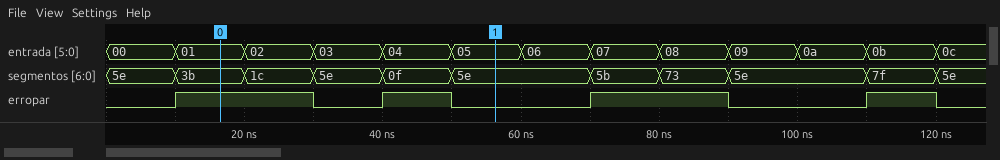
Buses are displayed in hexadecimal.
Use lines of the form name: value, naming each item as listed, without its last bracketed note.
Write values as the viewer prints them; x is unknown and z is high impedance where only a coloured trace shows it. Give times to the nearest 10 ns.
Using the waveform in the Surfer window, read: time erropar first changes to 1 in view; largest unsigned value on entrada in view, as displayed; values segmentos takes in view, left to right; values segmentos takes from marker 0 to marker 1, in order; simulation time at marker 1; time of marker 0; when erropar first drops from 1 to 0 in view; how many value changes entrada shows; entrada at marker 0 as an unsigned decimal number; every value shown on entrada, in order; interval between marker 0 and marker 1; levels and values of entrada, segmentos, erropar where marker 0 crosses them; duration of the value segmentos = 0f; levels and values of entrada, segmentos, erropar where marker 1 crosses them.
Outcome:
time erropar first changes to 1 in view: 10 ns
largest unsigned value on entrada in view, as displayed: 0c
values segmentos takes in view, left to right: 5e, 3b, 1c, 5e, 0f, 5e, 5b, 73, 5e, 7f, 5e
values segmentos takes from marker 0 to marker 1, in order: 3b, 1c, 5e, 0f, 5e
simulation time at marker 1: 60 ns
time of marker 0: 20 ns
when erropar first drops from 1 to 0 in view: 30 ns
how many value changes entrada shows: 12
entrada at marker 0 as an unsigned decimal number: 1
every value shown on entrada, in order: 00, 01, 02, 03, 04, 05, 06, 07, 08, 09, 0a, 0b, 0c
interval between marker 0 and marker 1: 40 ns
levels and values of entrada, segmentos, erropar where marker 0 crosses them: entrada=01, segmentos=3b, erropar=1
duration of the value segmentos = 0f: 10 ns
levels and values of entrada, segmentos, erropar where marker 1 crosses them: entrada=05, segmentos=5e, erropar=0
